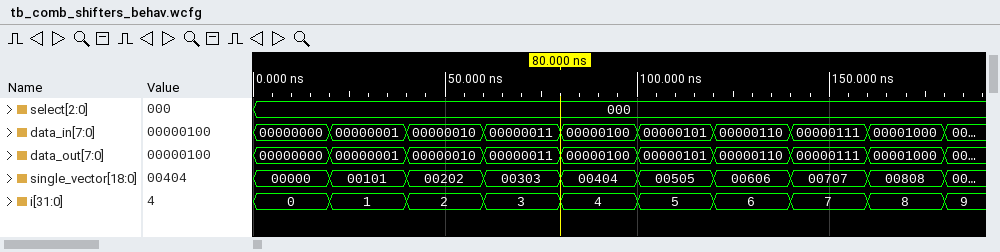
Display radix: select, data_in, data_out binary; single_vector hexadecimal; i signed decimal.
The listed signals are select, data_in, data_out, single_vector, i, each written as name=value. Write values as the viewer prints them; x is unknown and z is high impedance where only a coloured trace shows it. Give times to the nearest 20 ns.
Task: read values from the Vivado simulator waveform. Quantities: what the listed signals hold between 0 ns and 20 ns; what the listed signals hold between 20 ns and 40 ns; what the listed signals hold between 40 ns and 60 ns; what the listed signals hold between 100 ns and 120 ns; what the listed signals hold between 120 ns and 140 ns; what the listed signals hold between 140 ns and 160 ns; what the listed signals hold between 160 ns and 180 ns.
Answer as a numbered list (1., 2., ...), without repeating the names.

1. select=000, data_in=00000000, data_out=00000000, single_vector=00000, i=0
2. select=000, data_in=00000001, data_out=00000001, single_vector=00101, i=1
3. select=000, data_in=00000010, data_out=00000010, single_vector=00202, i=2
4. select=000, data_in=00000101, data_out=00000101, single_vector=00505, i=5
5. select=000, data_in=00000110, data_out=00000110, single_vector=00606, i=6
6. select=000, data_in=00000111, data_out=00000111, single_vector=00707, i=7
7. select=000, data_in=00001000, data_out=00001000, single_vector=00808, i=8
